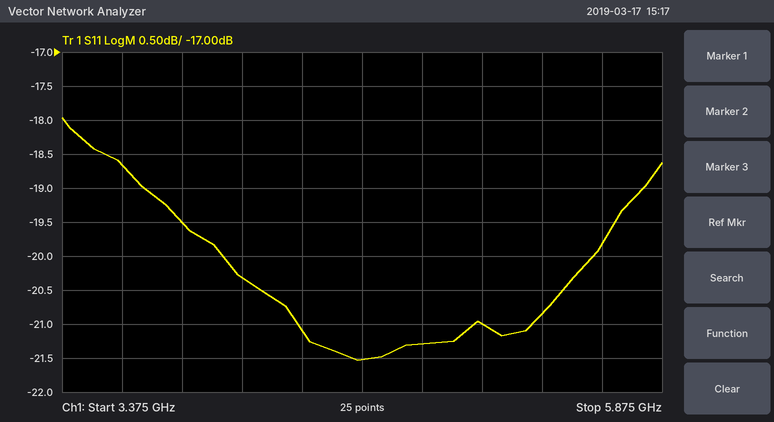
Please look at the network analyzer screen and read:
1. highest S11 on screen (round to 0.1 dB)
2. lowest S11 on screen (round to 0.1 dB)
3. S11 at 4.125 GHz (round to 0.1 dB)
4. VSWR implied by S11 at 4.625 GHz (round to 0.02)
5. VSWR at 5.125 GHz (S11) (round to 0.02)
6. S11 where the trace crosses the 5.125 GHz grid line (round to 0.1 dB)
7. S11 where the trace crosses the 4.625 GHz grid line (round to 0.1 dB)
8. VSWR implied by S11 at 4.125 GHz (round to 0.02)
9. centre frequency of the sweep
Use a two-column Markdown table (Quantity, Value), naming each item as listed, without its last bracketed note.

| Quantity | Value |
|---|---|
| highest S11 on screen | -18.0 dB |
| lowest S11 on screen | -21.5 dB |
| S11 at 4.125 GHz | -20.3 dB |
| VSWR implied by S11 at 4.625 GHz | 1.18 |
| VSWR at 5.125 GHz (S11) | 1.20 |
| S11 where the trace crosses the 5.125 GHz grid line | -21.0 dB |
| S11 where the trace crosses the 4.625 GHz grid line | -21.5 dB |
| VSWR implied by S11 at 4.125 GHz | 1.22 |
| centre frequency of the sweep | 4.625 GHz |
